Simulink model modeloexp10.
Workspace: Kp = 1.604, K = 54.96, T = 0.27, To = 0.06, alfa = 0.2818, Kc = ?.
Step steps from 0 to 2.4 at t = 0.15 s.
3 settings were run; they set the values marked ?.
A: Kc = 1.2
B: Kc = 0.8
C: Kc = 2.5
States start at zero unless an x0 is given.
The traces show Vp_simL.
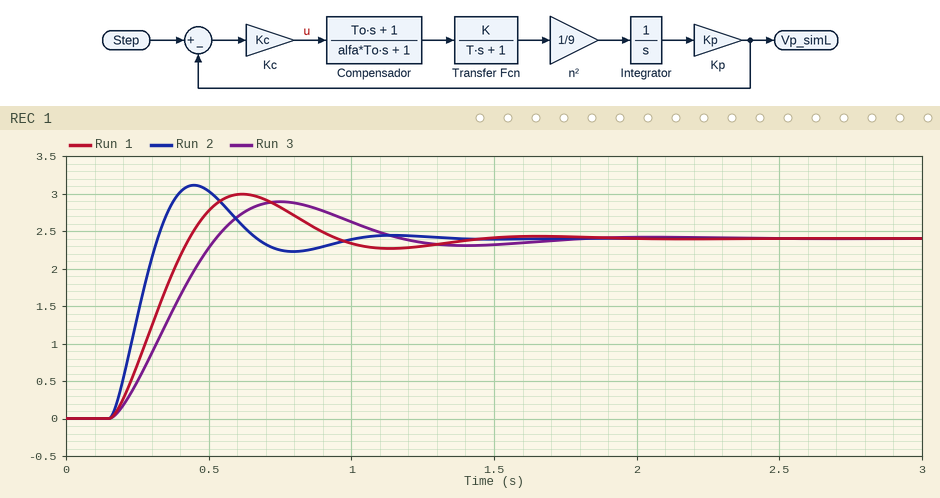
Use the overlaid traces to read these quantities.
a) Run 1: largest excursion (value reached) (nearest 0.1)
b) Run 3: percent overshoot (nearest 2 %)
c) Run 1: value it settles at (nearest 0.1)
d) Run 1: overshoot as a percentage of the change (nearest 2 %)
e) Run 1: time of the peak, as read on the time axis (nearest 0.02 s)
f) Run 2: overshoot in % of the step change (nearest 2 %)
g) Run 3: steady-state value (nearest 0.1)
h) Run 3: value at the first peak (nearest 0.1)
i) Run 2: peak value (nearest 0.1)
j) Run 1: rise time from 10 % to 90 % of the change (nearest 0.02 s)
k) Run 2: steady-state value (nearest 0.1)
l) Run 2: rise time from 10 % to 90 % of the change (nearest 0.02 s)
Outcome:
3.0
20 %
2.4
24 %
0.62 s
30 %
2.4
2.9
3.1
0.20 s
2.4
0.12 s
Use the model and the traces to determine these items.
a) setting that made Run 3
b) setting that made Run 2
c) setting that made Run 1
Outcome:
B
C
A
